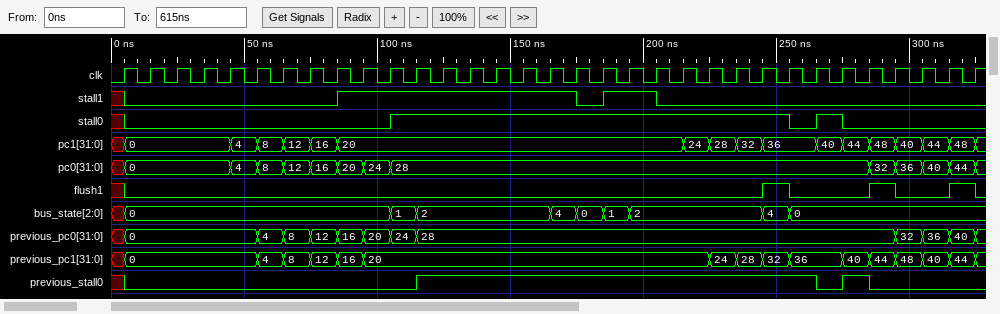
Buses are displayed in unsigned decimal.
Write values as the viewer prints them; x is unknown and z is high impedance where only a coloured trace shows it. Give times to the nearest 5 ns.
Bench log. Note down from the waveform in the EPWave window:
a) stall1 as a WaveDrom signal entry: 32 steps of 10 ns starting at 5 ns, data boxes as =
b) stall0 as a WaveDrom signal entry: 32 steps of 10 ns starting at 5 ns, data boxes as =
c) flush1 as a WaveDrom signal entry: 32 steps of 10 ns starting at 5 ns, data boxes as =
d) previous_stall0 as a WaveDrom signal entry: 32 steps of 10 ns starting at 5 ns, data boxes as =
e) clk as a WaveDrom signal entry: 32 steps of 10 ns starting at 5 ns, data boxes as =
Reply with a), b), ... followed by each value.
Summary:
a) {name: 'stall1', wave: '0.......1........01.0...........'}
b) {name: 'stall0', wave: '0.........1..............010....'}
c) {name: 'flush1', wave: '0.......................10..10.1'}
d) {name: 'previous_stall0', wave: '0..........1..............010...'}
e) {name: 'clk', wave: 'p...............................'}
